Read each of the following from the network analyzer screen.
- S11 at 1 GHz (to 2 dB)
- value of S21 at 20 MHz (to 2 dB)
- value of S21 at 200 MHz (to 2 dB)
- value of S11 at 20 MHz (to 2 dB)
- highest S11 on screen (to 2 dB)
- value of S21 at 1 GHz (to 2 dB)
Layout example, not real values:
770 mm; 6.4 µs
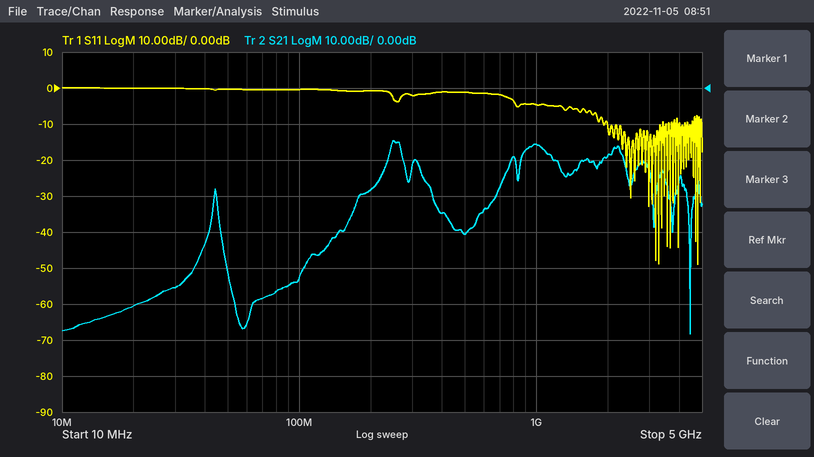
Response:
-4 dB; -60 dB; -28 dB; 0 dB; 0 dB; -16 dB
